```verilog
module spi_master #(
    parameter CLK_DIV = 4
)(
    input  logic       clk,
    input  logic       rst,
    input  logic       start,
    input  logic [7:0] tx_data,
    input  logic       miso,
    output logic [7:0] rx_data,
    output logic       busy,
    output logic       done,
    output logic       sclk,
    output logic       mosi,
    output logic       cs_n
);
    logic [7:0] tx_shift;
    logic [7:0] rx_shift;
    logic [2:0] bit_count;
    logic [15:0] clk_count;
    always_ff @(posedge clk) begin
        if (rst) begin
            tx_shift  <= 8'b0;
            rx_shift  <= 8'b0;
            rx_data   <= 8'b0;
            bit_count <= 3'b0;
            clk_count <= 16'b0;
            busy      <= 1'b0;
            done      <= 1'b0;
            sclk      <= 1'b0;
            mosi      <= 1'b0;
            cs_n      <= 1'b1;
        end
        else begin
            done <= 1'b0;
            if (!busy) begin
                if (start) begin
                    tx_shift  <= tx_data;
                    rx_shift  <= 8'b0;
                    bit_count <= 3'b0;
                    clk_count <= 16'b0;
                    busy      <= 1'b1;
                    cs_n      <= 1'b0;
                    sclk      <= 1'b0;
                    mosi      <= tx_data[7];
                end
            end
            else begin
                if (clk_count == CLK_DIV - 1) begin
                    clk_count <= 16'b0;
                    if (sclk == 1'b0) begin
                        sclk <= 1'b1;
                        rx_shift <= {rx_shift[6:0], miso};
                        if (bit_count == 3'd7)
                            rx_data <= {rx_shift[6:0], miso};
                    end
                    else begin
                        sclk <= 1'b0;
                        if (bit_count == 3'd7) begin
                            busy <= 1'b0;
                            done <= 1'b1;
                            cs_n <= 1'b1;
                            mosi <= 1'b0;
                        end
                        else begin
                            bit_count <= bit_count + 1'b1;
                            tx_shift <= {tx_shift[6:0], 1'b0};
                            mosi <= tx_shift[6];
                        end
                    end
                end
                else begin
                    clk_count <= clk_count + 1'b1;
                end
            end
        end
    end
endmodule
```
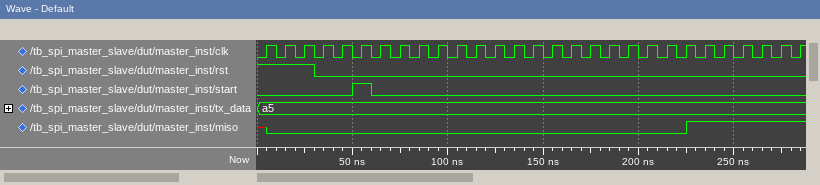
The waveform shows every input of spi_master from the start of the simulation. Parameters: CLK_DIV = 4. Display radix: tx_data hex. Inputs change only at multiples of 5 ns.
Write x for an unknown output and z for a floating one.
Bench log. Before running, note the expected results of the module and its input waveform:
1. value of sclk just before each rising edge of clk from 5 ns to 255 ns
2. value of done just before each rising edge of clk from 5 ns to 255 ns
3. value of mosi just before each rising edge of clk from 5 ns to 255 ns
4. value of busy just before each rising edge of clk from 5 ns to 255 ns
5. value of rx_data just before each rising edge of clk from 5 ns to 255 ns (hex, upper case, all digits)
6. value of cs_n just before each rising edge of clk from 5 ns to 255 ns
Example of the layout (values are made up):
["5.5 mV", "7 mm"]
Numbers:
["x 0 0 0 0 0 0 0 0 0 1 1 1 1 0 0 0 0 1 1 1 1 0 0 0 0", "x 0 0 0 0 0 0 0 0 0 0 0 0 0 0 0 0 0 0 0 0 0 0 0 0 0", "x 0 0 0 0 0 1 1 1 1 1 1 1 1 0 0 0 0 0 0 0 0 1 1 1 1", "x 0 0 0 0 0 1 1 1 1 1 1 1 1 1 1 1 1 1 1 1 1 1 1 1 1", "x, 00, 00, 00, 00, 00, 00, 00, 00, 00, 00, 00, 00, 00, 00, 00, 00, 00, 00, 00, 00, 00, 00, 00, 00, 00", "x 1 1 1 1 1 0 0 0 0 0 0 0 0 0 0 0 0 0 0 0 0 0 0 0 0"]
